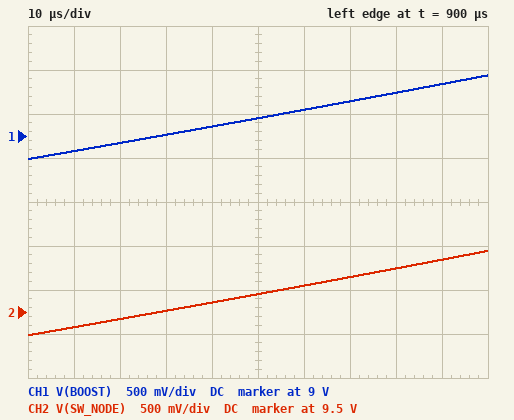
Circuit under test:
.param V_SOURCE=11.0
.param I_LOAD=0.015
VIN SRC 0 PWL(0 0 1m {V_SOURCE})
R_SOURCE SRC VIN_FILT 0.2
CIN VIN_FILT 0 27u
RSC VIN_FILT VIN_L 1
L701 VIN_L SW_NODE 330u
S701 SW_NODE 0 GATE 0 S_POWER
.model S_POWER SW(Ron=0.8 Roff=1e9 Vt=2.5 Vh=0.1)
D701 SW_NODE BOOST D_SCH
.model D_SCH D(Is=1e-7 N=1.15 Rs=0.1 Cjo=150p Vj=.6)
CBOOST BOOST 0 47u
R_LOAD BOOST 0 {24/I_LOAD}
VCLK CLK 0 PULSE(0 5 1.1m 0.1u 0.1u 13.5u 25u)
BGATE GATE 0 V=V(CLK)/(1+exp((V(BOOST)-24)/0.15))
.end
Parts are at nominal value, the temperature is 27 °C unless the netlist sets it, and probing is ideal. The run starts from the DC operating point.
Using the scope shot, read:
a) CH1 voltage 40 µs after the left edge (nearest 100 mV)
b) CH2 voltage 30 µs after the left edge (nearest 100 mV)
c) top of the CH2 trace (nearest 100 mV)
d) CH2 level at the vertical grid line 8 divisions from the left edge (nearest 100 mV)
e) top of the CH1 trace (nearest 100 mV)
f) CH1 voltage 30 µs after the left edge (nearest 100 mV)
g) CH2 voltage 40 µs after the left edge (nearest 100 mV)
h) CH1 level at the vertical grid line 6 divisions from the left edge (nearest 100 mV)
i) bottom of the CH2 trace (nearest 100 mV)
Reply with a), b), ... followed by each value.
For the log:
a) 9.1 V
b) 9.5 V
c) 10.2 V
d) 10.0 V
e) 9.7 V
f) 9.0 V
g) 9.6 V
h) 9.3 V
i) 9.2 V
